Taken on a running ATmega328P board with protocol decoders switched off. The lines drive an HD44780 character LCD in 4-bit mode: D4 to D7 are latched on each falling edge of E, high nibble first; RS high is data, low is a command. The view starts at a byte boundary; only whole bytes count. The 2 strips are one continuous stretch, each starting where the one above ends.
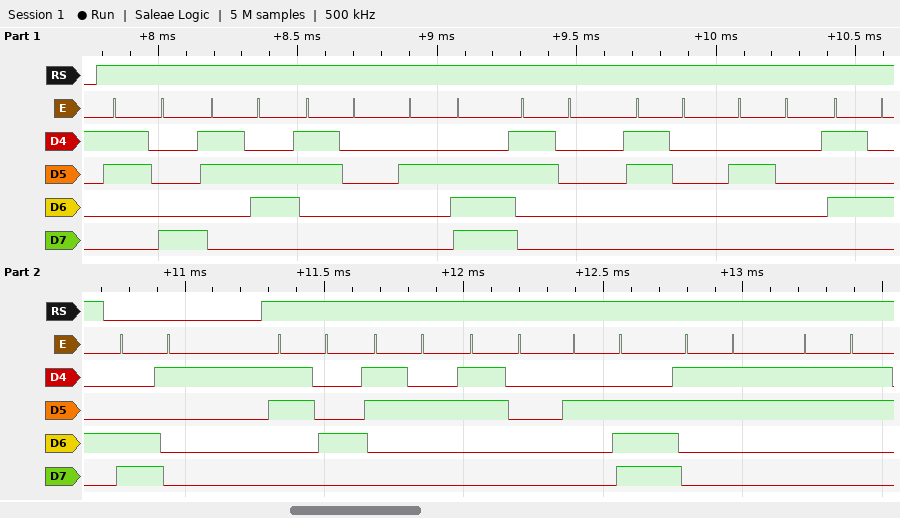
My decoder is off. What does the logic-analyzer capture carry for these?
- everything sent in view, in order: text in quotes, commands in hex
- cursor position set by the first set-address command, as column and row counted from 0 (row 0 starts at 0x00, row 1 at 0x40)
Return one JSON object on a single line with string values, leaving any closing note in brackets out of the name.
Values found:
{"everything sent in view, in order: text in quotes, commands in hex": "\"860.00 T\" 0xC1 \"420.33\"", "cursor position set by the first set-address command, as column and row counted from 0": "column 1, row 1"}
